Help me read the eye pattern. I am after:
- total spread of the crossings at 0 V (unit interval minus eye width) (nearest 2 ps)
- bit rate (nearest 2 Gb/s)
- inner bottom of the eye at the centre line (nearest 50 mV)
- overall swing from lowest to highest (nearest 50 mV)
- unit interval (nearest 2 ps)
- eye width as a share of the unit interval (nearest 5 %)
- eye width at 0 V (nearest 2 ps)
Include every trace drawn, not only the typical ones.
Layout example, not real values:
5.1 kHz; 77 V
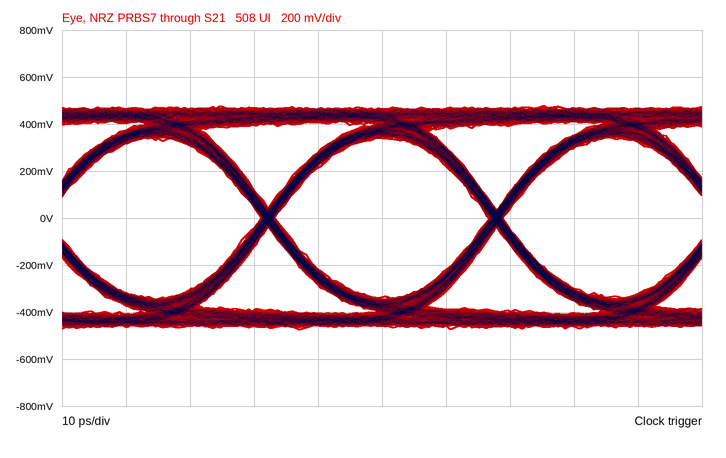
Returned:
2 ps; 28 Gb/s; -350 mV; 950 mV; 36 ps; 95 %; 34 ps
